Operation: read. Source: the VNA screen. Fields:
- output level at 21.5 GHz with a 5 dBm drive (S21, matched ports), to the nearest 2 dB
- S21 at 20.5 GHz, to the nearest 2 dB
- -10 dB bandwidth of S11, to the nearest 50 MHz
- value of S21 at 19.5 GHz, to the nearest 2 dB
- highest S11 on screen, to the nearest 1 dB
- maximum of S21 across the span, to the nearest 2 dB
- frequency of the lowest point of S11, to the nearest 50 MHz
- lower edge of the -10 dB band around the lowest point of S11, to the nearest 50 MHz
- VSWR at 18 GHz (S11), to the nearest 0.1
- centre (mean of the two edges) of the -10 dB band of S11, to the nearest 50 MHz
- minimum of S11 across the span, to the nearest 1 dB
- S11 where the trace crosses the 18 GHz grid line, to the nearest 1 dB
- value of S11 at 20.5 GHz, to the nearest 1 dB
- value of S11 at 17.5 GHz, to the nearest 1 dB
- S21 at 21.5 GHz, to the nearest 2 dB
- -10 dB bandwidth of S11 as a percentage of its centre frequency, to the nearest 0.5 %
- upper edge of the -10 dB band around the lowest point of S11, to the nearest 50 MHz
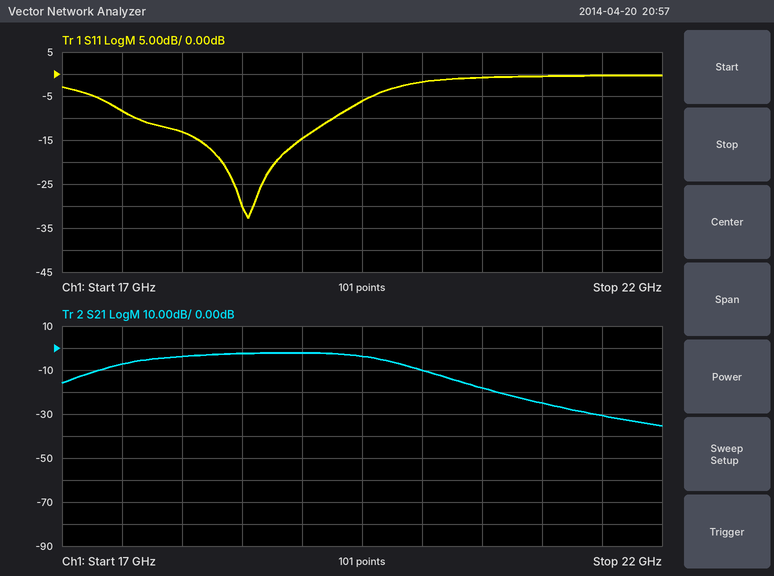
-26 dBm
-18 dB
1.65 GHz
-4 dB
0 dB
-2 dB
18.55 GHz
17.60 GHz
1.6
18.45 GHz
-33 dB
-13 dB
-1 dB
-8 dB
-30 dB
9.0 %
19.25 GHz
